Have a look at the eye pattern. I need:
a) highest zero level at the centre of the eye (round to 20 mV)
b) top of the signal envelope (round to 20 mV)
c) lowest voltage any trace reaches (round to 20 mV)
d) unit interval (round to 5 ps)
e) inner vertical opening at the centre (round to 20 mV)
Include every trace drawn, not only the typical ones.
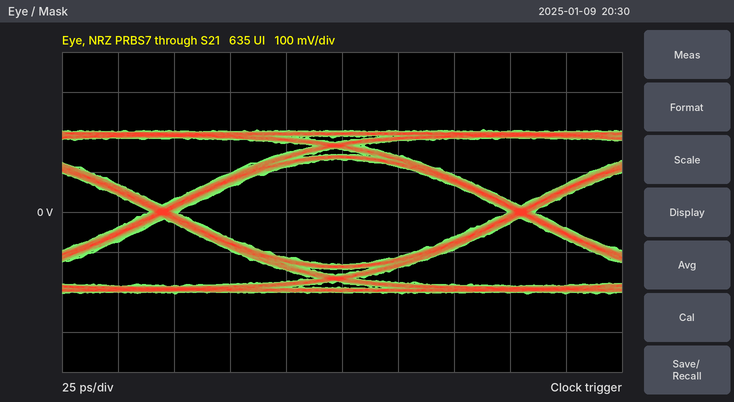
-140 mV
200 mV
-200 mV
160 ps
260 mV
